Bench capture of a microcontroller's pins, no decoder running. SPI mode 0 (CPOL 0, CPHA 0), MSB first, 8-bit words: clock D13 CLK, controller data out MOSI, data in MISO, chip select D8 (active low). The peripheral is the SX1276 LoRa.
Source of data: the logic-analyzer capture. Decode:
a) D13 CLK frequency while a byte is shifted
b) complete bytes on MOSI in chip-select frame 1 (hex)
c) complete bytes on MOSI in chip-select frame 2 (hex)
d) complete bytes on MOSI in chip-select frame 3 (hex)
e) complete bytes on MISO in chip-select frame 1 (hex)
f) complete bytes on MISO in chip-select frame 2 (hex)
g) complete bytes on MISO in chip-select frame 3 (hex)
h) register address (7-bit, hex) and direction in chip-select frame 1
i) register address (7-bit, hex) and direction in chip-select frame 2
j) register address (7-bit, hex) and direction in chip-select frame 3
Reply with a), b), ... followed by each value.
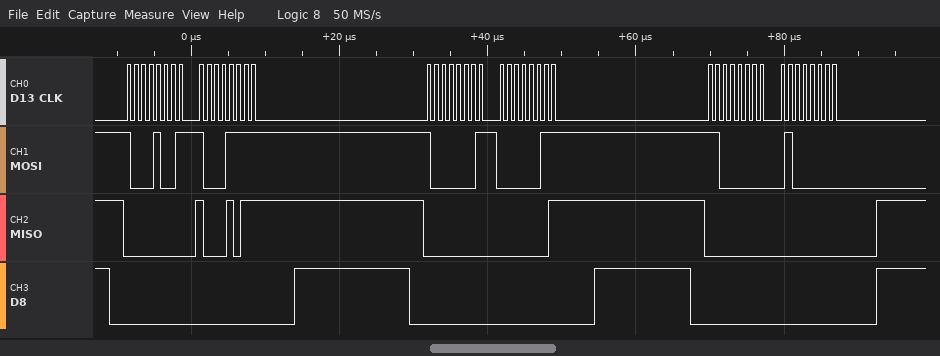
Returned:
a) 1 MHz
b) 89 8F
c) 81 03
d) C0 40
e) 00 8B
f) 00 01
g) 00 00
h) 0x09 write
i) 0x01 write
j) 0x40 write
